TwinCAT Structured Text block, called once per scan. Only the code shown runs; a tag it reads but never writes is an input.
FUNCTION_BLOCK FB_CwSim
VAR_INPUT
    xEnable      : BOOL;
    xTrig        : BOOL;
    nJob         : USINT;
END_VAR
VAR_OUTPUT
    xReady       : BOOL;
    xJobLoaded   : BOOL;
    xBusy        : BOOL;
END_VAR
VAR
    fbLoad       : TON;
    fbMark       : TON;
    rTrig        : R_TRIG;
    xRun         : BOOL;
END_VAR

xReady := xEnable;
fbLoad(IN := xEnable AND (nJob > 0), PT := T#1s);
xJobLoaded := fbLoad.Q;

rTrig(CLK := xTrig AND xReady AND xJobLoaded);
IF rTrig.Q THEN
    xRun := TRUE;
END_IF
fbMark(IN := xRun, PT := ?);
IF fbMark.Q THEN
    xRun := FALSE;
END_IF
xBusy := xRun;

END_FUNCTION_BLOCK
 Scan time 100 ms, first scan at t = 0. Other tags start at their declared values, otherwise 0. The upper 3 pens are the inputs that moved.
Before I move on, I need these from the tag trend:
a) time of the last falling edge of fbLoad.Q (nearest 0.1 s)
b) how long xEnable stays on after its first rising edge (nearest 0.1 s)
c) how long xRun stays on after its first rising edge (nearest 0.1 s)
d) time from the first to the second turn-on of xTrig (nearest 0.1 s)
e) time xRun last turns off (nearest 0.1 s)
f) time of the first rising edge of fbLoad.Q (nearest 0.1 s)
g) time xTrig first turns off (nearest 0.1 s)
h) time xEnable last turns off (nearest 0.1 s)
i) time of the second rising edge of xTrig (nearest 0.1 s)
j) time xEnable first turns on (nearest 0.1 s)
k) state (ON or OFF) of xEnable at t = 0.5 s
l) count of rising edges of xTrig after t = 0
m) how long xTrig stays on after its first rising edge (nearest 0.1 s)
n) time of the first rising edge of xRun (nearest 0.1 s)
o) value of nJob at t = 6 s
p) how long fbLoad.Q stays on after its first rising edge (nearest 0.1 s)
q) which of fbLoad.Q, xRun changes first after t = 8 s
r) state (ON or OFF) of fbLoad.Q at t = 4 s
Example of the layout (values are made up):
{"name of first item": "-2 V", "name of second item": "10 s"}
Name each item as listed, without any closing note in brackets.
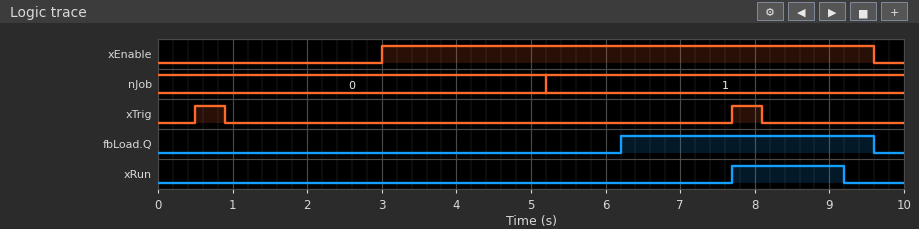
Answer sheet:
{"time of the last falling edge of fbLoad.Q": "9.6 s", "how long xEnable stays on after its first rising edge": "6.6 s", "how long xRun stays on after its first rising edge": "1.5 s", "time from the first to the second turn-on of xTrig": "7.2 s", "time xRun last turns off": "9.2 s", "time of the first rising edge of fbLoad.Q": "6.2 s", "time xTrig first turns off": "0.9 s", "time xEnable last turns off": "9.6 s", "time of the second rising edge of xTrig": "7.7 s", "time xEnable first turns on": "3.0 s", "state (ON or OFF) of xEnable at t = 0.5 s": "OFF", "count of rising edges of xTrig after t = 0": "2", "how long xTrig stays on after its first rising edge": "0.4 s", "time of the first rising edge of xRun": "7.7 s", "value of nJob at t = 6 s": "1", "how long fbLoad.Q stays on after its first rising edge": "3.4 s", "which of fbLoad.Q, xRun changes first after t = 8 s": "xRun", "state (ON or OFF) of fbLoad.Q at t = 4 s": "OFF"}
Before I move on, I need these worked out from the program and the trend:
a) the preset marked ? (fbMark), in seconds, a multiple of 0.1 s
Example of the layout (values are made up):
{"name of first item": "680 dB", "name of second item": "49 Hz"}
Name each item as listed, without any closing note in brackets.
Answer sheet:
{"the preset marked ? (fbMark), in seconds, a multiple of 0.1 s": "1.5 s"}
